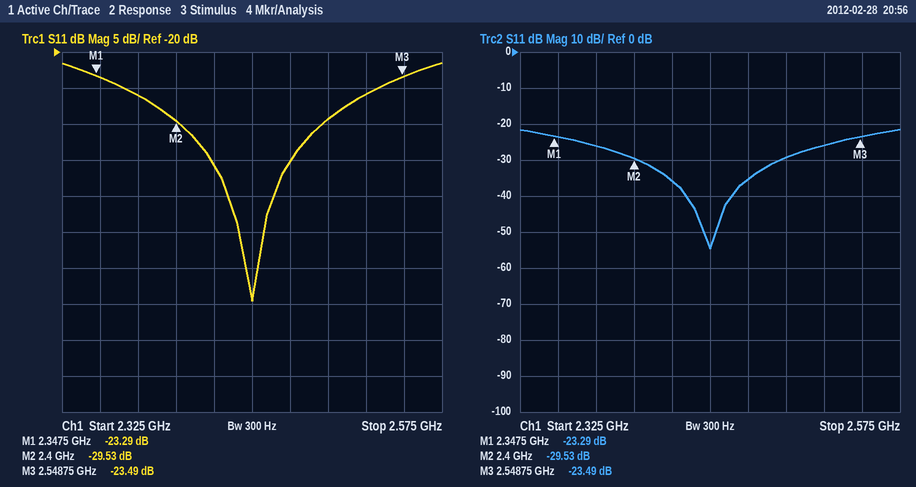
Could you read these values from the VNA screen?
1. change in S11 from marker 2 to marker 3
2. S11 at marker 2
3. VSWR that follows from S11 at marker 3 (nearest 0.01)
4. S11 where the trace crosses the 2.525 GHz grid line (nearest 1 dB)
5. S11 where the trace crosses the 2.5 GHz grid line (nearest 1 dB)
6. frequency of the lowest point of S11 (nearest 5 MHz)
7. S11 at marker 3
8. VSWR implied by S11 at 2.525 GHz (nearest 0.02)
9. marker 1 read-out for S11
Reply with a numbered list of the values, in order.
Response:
1. 6.04 dB
2. -29.53 dB
3. 1.14
4. -26 dB
5. -29 dB
6. 2.450 GHz
7. -23.49 dB
8. 1.10
9. -23.29 dB
